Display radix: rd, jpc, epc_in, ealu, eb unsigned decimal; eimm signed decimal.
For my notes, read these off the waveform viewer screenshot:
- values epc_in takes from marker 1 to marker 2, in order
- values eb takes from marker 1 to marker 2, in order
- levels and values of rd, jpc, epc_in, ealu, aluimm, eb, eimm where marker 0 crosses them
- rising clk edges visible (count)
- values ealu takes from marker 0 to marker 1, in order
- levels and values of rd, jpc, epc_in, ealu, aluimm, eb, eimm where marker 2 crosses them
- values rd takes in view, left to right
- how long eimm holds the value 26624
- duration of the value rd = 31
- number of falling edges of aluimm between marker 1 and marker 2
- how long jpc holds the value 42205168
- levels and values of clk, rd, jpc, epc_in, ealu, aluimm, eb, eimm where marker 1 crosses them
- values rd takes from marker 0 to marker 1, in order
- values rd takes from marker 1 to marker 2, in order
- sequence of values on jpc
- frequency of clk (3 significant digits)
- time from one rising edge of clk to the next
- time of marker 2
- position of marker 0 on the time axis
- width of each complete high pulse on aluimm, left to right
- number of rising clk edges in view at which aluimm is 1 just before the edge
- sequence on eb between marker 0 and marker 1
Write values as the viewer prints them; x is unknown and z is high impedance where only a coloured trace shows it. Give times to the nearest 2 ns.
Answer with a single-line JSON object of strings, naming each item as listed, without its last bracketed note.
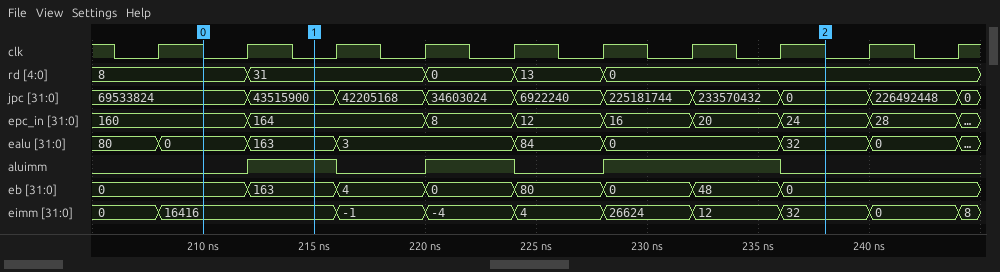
{"values epc_in takes from marker 1 to marker 2, in order": "164, 8, 12, 16, 20, 24", "values eb takes from marker 1 to marker 2, in order": "163, 4, 0, 80, 0, 48, 0", "levels and values of rd, jpc, epc_in, ealu, aluimm, eb, eimm where marker 0 crosses them": "rd=8, jpc=69533824, epc_in=160, ealu=0, aluimm=0, eb=0, eimm=16416", "rising clk edges visible": "10", "values ealu takes from marker 0 to marker 1, in order": "0, 163", "levels and values of rd, jpc, epc_in, ealu, aluimm, eb, eimm where marker 2 crosses them": "rd=0, jpc=0, epc_in=24, ealu=32, aluimm=0, eb=0, eimm=32", "values rd takes in view, left to right": "8, 31, 0, 13, 0", "how long eimm holds the value 26624": "4 ns", "duration of the value rd = 31": "8 ns", "number of falling edges of aluimm between marker 1 and marker 2": "3", "how long jpc holds the value 42205168": "4 ns", "levels and values of clk, rd, jpc, epc_in, ealu, aluimm, eb, eimm where marker 1 crosses them": "clk=0, rd=31, jpc=43515900, epc_in=164, ealu=163, aluimm=1, eb=163, eimm=16416", "values rd takes from marker 0 to marker 1, in order": "8, 31", "values rd takes from marker 1 to marker 2, in order": "31, 0, 13, 0", "sequence of values on jpc": "69533824, 43515900, 42205168, 34603024, 6922240, 225181744, 233570432, 0, 226492448, 0", "frequency of clk": "250 MHz", "time from one rising edge of clk to the next": "4 ns", "time of marker 2": "238 ns", "position of marker 0 on the time axis": "210 ns", "width of each complete high pulse on aluimm, left to right": "4 ns, 4 ns, 8 ns", "number of rising clk edges in view at which aluimm is 1 just before the edge": "4", "sequence on eb between marker 0 and marker 1": "0, 163"}
